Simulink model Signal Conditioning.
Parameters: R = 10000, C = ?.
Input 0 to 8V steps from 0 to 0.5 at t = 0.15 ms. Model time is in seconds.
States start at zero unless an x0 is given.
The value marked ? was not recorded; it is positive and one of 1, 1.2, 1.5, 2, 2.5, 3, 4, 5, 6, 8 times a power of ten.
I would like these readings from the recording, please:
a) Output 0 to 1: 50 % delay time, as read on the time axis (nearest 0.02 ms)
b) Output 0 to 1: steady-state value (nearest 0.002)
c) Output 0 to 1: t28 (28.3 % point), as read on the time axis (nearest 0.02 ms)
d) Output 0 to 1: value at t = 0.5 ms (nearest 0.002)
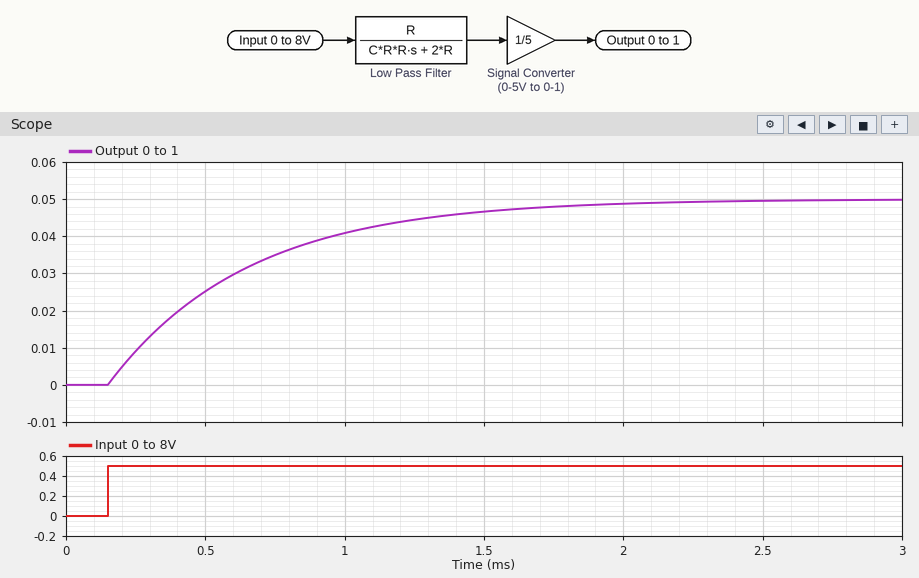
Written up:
0.50 ms
0.050
0.32 ms
0.026
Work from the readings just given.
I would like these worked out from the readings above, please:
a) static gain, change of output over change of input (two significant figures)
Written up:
0.10
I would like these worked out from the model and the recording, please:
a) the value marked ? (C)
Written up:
1e-07
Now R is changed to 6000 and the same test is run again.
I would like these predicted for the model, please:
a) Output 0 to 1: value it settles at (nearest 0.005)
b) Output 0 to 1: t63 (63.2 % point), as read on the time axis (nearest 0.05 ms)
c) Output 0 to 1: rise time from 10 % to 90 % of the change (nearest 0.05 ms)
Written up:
0.050
0.45 ms
0.65 ms
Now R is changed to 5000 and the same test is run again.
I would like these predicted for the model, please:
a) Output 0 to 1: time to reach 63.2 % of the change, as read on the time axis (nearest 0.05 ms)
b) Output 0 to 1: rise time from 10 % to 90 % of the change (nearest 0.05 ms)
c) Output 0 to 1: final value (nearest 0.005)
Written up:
0.40 ms
0.55 ms
0.050
